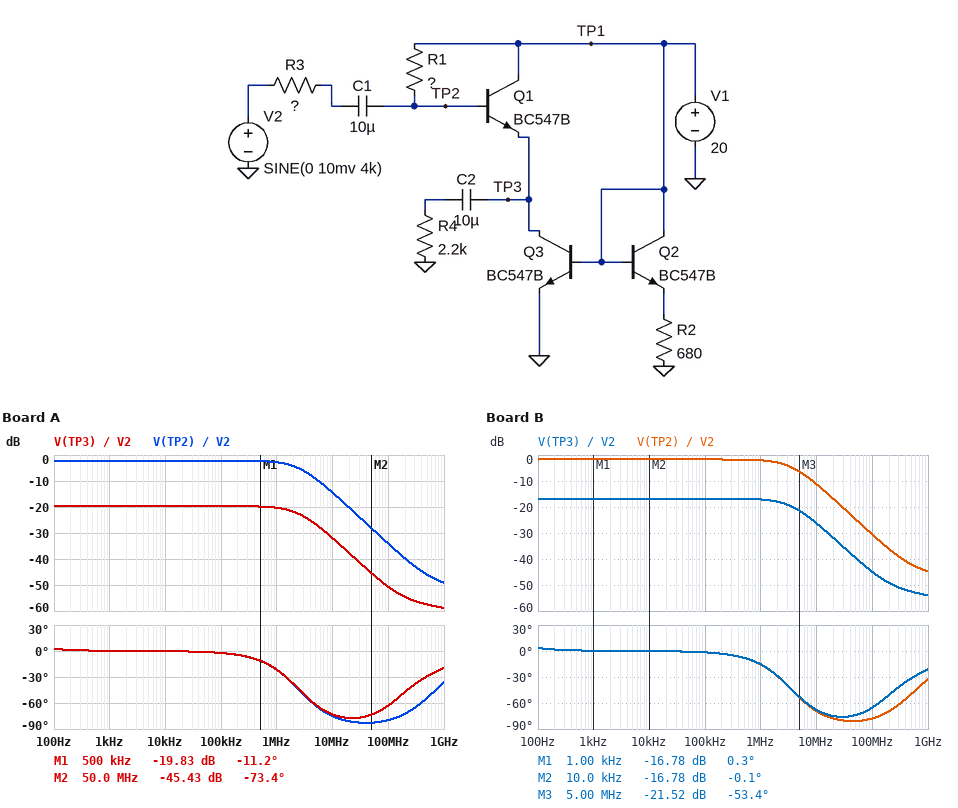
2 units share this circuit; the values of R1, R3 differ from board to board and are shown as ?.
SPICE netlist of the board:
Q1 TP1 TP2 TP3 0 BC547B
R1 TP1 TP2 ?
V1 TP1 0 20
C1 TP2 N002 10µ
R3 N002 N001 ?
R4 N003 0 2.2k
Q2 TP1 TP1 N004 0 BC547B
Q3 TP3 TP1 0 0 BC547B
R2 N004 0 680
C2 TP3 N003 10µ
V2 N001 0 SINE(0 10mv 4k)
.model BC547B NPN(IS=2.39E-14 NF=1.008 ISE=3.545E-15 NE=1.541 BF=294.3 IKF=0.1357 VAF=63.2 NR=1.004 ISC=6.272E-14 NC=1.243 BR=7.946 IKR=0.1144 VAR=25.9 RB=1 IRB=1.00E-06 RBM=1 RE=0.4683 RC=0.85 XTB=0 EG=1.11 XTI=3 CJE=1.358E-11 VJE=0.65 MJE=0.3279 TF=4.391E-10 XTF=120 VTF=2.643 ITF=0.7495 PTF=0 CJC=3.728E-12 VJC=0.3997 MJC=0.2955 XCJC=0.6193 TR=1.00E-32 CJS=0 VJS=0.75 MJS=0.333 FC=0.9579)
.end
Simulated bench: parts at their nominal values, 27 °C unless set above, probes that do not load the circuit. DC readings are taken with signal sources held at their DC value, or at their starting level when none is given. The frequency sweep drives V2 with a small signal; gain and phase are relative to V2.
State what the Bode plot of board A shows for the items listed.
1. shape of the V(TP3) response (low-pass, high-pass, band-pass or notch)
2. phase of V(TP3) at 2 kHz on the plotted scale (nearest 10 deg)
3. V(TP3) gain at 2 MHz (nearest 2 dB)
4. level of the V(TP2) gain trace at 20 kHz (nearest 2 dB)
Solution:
low-pass
0 deg
-22 dB
-2 dB
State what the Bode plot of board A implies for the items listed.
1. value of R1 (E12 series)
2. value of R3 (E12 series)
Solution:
1.2 MΩ
820 Ω
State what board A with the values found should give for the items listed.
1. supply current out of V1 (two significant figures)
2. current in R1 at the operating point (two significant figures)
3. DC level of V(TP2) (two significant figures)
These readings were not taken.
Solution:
13 A
11 µA
6.8 V
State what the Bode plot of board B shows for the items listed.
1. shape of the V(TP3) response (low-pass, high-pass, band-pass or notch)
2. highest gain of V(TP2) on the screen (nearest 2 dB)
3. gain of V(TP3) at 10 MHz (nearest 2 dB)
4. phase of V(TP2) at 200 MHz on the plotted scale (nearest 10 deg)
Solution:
low-pass
-2 dB
-26 dB
-70 deg
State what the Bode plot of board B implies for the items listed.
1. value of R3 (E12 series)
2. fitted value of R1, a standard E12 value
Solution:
470 Ω
820 kΩ
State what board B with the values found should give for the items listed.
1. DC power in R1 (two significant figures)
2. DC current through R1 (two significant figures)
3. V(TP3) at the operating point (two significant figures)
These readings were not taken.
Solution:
210 µW
16 µA
6.1 V
